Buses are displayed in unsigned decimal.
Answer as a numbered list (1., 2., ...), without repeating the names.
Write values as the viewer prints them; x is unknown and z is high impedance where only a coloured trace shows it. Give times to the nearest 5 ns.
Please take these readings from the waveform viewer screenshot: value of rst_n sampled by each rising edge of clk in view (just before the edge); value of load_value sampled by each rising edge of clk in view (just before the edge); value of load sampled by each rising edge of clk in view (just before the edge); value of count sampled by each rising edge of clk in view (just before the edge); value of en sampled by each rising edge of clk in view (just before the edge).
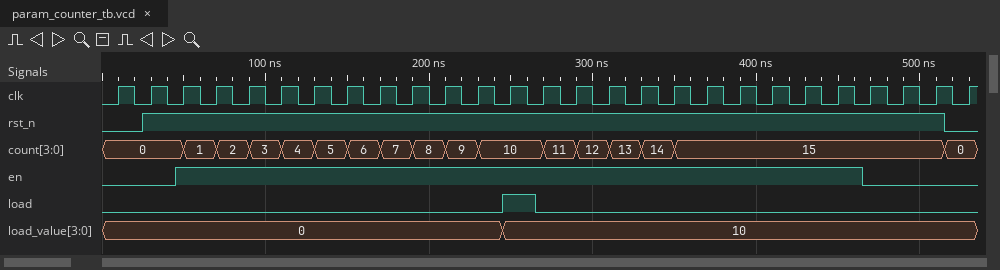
1. 0 1 1 1 1 1 1 1 1 1 1 1 1 1 1 1 1 1 1 1 1 1 1 1 1 1 0
2. 0, 0, 0, 0, 0, 0, 0, 0, 0, 0, 0, 0, 10, 10, 10, 10, 10, 10, 10, 10, 10, 10, 10, 10, 10, 10, 10
3. 0 0 0 0 0 0 0 0 0 0 0 0 1 0 0 0 0 0 0 0 0 0 0 0 0 0 0
4. 0, 0, 0, 1, 2, 3, 4, 5, 6, 7, 8, 9, 10, 10, 11, 12, 13, 14, 15, 15, 15, 15, 15, 15, 15, 15, 0
5. 0 0 1 1 1 1 1 1 1 1 1 1 1 1 1 1 1 1 1 1 1 1 1 0 0 0 0
